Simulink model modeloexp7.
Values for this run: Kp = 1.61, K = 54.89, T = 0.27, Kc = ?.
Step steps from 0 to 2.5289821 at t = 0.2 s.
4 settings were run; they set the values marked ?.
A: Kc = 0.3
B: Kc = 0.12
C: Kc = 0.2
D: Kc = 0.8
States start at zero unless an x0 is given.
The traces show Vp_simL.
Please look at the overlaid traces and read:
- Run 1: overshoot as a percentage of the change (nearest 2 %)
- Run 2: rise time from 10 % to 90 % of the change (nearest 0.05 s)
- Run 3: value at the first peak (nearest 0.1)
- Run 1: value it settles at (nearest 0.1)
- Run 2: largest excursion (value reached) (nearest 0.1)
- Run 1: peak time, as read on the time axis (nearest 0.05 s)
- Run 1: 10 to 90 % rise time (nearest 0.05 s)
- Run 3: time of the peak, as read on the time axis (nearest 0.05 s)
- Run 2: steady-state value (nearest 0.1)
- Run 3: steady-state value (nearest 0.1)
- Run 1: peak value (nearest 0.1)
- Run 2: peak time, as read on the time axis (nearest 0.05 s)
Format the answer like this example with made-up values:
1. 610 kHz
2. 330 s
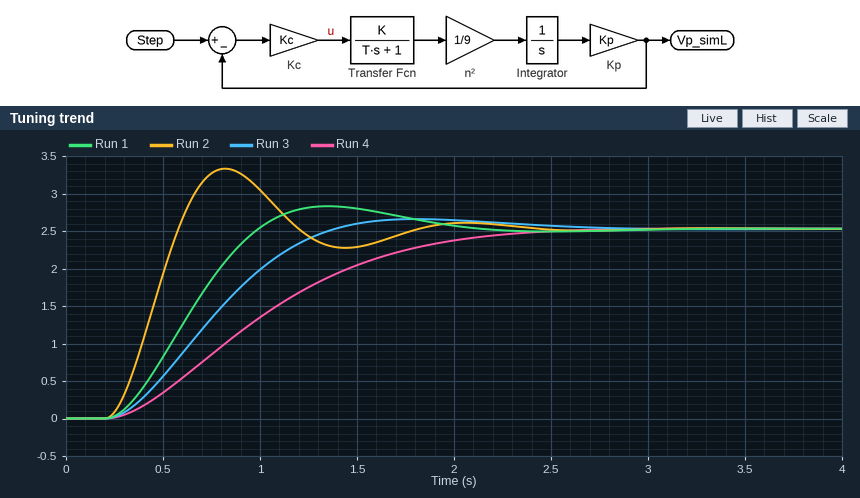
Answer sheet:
1. 12 %
2. 0.25 s
3. 2.7
4. 2.5
5. 3.3
6. 1.35 s
7. 0.55 s
8. 1.80 s
9. 2.5
10. 2.5
11. 2.8
12. 0.80 s
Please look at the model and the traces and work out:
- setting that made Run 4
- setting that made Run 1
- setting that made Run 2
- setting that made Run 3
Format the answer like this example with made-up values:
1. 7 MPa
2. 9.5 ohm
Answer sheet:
1. B
2. A
3. D
4. C
